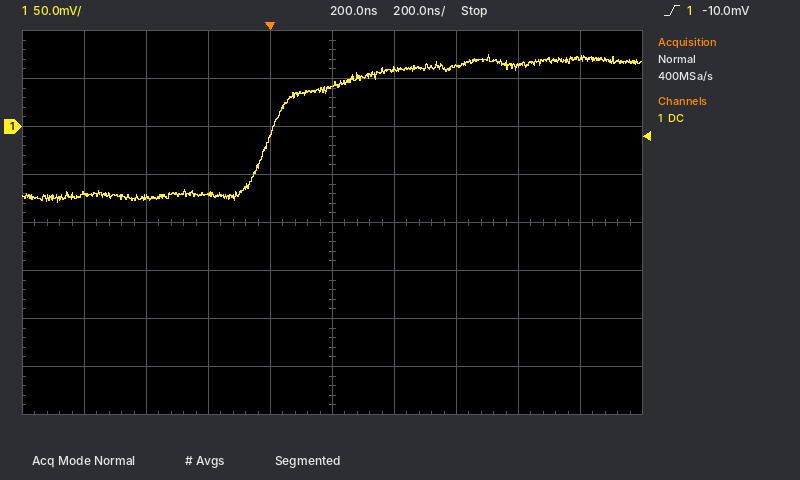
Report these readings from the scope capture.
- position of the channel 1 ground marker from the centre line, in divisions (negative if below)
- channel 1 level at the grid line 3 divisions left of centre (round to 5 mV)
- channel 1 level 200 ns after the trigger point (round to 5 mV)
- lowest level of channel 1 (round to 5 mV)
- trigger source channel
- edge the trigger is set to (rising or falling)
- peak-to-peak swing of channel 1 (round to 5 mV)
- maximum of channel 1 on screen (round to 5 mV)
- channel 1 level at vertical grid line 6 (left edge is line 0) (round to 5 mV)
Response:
+2.0 div
-75 mV
45 mV
-80 mV
channel 1
rising
155 mV
75 mV
60 mV
